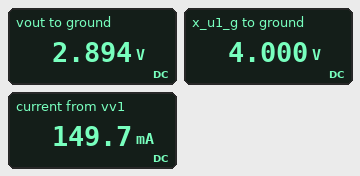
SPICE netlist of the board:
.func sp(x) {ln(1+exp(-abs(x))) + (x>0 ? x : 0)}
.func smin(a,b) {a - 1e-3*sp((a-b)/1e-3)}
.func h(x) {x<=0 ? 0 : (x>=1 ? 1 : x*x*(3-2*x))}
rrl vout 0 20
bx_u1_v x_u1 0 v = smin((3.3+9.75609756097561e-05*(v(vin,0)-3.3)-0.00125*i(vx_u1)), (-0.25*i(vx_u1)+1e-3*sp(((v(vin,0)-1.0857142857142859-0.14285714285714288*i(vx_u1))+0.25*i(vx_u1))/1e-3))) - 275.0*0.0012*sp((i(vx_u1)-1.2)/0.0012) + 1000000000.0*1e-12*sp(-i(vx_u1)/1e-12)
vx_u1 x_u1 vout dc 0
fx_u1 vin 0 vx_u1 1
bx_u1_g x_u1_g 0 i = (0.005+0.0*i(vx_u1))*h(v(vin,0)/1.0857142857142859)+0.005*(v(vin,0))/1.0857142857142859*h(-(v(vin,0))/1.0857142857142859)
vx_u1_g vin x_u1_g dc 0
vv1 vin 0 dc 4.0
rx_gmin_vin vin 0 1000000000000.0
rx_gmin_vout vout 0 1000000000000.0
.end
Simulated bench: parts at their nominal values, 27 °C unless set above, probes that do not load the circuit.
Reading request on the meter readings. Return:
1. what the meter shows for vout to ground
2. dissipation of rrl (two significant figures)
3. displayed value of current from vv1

2.894 V
420 mW
149.7 mA
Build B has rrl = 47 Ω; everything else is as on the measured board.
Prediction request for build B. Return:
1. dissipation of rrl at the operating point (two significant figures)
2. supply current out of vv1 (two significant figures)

180 mW
67 mA
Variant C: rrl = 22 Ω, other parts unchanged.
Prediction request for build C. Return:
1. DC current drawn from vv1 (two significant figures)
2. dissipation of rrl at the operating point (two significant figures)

140 mA
380 mW
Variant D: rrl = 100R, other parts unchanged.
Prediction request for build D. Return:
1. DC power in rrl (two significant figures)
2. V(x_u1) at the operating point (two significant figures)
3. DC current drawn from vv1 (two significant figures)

85 mW
2.9 V
34 mA
